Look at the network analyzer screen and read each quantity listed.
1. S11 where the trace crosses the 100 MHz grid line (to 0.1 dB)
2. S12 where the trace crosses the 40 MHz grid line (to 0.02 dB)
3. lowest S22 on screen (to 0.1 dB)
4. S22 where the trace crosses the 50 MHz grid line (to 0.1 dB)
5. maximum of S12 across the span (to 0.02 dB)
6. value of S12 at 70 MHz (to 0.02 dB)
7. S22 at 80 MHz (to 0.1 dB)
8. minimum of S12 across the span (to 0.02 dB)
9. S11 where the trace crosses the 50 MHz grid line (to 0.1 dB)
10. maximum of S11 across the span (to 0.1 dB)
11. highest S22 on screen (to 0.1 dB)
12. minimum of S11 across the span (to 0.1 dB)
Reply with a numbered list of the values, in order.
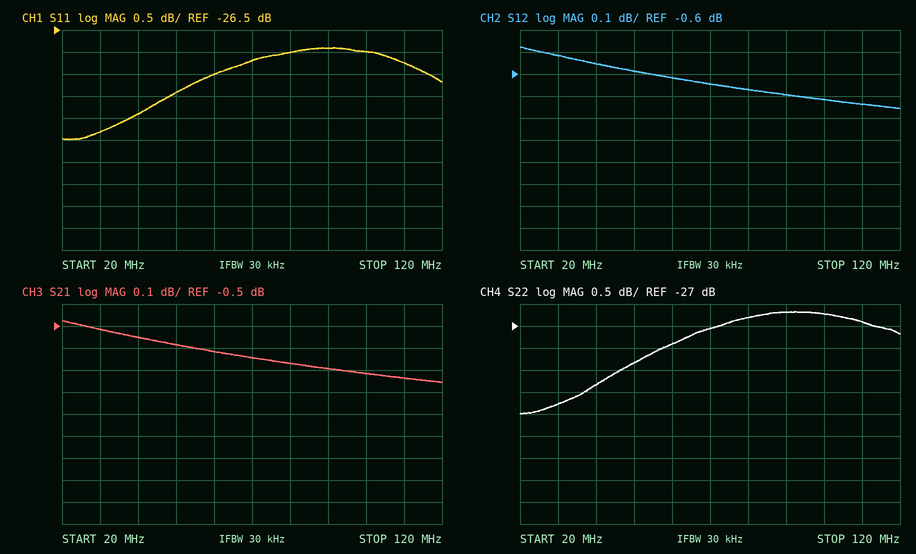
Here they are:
1. -27.0 dB
2. -0.56 dB
3. -29.0 dB
4. -27.8 dB
5. -0.48 dB
6. -0.64 dB
7. -26.8 dB
8. -0.76 dB
9. -27.9 dB
10. -26.9 dB
11. -26.7 dB
12. -29.0 dB
